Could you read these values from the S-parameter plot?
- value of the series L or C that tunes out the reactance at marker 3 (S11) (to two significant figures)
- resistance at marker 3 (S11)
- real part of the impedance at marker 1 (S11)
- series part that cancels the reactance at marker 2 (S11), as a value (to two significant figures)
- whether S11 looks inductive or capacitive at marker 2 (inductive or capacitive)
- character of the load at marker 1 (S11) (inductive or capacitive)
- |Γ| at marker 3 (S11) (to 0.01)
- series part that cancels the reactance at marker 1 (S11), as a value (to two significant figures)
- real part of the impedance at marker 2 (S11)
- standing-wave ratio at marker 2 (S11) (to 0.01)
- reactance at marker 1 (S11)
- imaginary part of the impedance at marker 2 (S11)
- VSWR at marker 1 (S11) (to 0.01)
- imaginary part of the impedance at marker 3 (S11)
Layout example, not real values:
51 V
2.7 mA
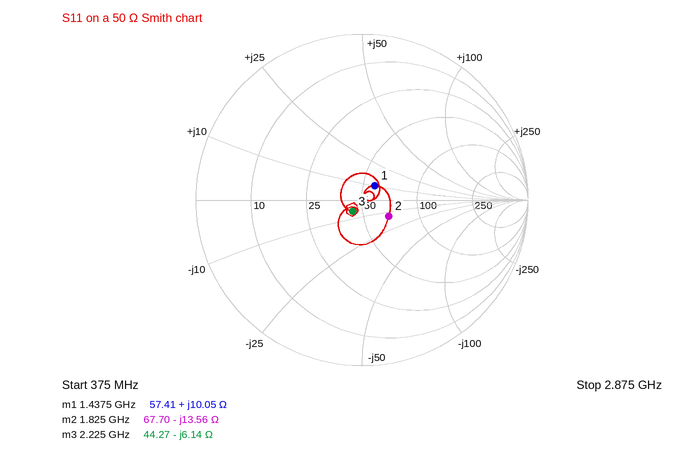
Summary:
440 pH
44.27 Ω
57.41 Ω
1.2 nH
capacitive
inductive
0.09
11 pF
67.70 Ω
1.46
+10.05 Ω
-13.56 Ω
1.26
-6.14 Ω
